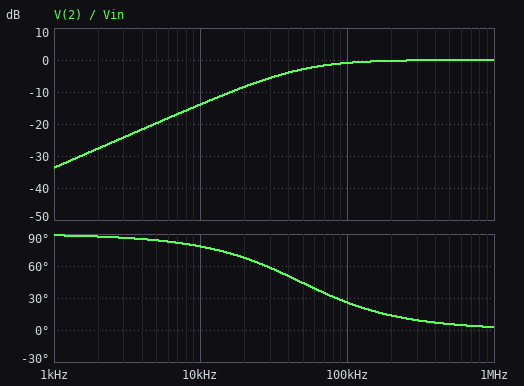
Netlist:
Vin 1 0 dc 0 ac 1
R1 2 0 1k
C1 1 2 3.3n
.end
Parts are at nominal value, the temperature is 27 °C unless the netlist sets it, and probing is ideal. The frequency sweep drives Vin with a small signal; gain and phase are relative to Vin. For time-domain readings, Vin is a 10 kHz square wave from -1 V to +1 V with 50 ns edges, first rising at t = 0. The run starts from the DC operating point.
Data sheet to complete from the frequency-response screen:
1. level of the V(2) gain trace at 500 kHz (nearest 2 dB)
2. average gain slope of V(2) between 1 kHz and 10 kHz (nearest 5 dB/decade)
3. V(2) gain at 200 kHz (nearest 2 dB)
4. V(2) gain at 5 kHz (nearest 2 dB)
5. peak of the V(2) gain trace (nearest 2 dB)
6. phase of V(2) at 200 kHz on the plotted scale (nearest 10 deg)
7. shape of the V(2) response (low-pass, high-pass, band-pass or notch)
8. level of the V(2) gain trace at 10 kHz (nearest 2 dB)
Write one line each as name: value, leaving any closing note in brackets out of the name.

level of the V(2) gain trace at 500 kHz: 0 dB
average gain slope of V(2) between 1 kHz and 10 kHz: 20 dB/decade
V(2) gain at 200 kHz: 0 dB
V(2) gain at 5 kHz: -20 dB
peak of the V(2) gain trace: 0 dB
phase of V(2) at 200 kHz on the plotted scale: 10 deg
shape of the V(2) response: high-pass
level of the V(2) gain trace at 10 kHz: -14 dB
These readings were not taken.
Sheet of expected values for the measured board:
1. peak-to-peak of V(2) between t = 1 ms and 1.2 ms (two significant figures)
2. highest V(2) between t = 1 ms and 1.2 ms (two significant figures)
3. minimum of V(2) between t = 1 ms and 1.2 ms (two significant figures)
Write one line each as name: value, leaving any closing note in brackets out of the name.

peak-to-peak of V(2) between t = 1 ms and 1.2 ms: 4.0 V
highest V(2) between t = 1 ms and 1.2 ms: 2.0 V
minimum of V(2) between t = 1 ms and 1.2 ms: -2.0 V
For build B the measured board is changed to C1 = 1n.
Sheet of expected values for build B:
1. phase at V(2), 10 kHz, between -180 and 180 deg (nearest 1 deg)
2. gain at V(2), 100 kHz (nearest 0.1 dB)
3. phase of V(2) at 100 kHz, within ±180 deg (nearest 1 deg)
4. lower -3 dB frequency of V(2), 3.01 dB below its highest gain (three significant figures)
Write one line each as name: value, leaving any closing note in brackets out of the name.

phase at V(2), 10 kHz, between -180 and 180 deg: 86 deg
gain at V(2), 100 kHz: -5.5 dB
phase of V(2) at 100 kHz, within ±180 deg: 58 deg
lower -3 dB frequency of V(2), 3.01 dB below its highest gain: 159 kHz
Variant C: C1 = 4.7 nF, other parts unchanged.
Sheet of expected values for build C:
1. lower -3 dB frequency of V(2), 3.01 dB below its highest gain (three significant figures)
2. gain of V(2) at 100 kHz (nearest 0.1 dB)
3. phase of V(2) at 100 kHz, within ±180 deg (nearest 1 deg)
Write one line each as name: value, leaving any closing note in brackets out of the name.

lower -3 dB frequency of V(2), 3.01 dB below its highest gain: 33.9 kHz
gain of V(2) at 100 kHz: -0.5 dB
phase of V(2) at 100 kHz, within ±180 deg: 19 deg
